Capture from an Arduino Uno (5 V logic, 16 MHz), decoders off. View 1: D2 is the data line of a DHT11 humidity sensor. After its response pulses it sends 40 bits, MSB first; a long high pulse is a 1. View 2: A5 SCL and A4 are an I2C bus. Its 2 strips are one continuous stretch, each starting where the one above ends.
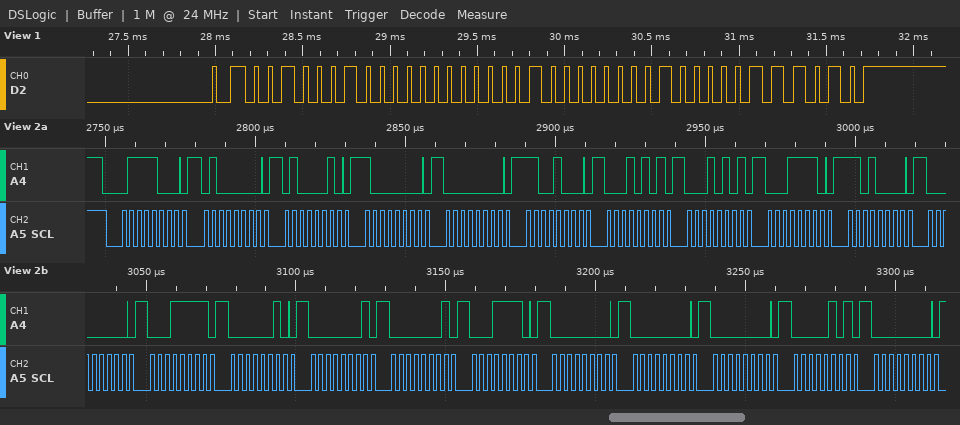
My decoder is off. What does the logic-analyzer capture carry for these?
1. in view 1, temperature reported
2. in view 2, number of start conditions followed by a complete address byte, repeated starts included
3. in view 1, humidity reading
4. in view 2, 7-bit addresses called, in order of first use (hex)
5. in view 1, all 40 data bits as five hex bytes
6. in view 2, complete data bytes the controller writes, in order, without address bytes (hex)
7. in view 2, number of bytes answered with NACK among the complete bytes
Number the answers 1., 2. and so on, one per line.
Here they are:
1. 16.8 °C
2. 1
3. 34 %
4. 0x3C
5. 22 00 10 08 3A
6. 40 42 80 00 C8 15 15 1E D0 00 1F 02 01 01 1E 00 00 00 05 00
7. 0
